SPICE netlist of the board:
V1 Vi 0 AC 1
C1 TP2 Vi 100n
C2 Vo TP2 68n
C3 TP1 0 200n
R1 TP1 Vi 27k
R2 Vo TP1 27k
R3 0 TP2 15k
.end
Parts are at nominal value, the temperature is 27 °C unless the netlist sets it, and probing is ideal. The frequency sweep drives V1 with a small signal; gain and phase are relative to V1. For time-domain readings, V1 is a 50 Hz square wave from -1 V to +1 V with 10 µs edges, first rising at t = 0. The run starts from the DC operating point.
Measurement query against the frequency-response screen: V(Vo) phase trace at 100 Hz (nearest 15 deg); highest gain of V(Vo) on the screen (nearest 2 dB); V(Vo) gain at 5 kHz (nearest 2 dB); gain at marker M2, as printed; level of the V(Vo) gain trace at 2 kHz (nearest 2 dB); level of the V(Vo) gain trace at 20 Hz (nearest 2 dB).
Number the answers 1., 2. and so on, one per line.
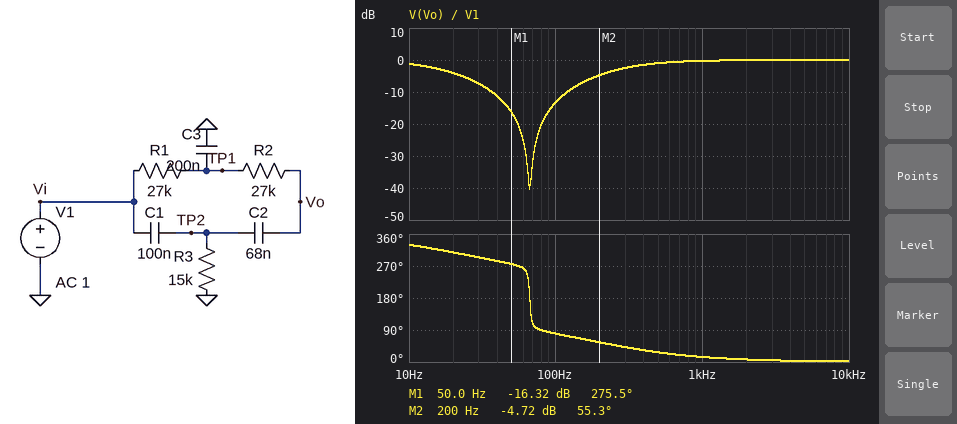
1. 75 deg
2. 0 dB
3. 0 dB
4. -4.72 dB
5. 0 dB
6. -4 dB
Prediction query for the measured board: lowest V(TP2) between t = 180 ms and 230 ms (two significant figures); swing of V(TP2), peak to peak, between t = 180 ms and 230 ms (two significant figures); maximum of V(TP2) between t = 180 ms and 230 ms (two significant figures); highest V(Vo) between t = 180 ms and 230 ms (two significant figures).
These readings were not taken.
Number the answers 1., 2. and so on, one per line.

1. -1.9 V
2. 3.8 V
3. 1.9 V
4. 1.5 V
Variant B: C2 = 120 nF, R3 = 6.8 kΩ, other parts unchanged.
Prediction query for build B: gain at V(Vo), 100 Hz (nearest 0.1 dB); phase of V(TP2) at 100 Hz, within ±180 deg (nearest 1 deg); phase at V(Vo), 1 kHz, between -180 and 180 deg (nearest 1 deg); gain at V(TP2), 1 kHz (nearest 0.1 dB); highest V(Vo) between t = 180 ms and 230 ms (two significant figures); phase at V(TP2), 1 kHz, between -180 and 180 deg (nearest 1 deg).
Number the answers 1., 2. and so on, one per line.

1. -15.1 dB
2. 59 deg
3. 19 deg
4. -0.4 dB
5. 1.6 V
6. 16 deg
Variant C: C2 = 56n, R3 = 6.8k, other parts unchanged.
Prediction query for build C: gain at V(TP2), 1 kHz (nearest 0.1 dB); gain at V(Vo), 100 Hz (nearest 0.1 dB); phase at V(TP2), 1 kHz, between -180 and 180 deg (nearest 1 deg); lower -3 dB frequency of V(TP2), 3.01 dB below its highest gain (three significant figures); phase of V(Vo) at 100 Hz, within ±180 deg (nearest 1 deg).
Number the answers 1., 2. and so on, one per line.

1. -0.4 dB
2. -19.6 dB
3. 16 deg
4. 316 Hz
5. 146 deg
